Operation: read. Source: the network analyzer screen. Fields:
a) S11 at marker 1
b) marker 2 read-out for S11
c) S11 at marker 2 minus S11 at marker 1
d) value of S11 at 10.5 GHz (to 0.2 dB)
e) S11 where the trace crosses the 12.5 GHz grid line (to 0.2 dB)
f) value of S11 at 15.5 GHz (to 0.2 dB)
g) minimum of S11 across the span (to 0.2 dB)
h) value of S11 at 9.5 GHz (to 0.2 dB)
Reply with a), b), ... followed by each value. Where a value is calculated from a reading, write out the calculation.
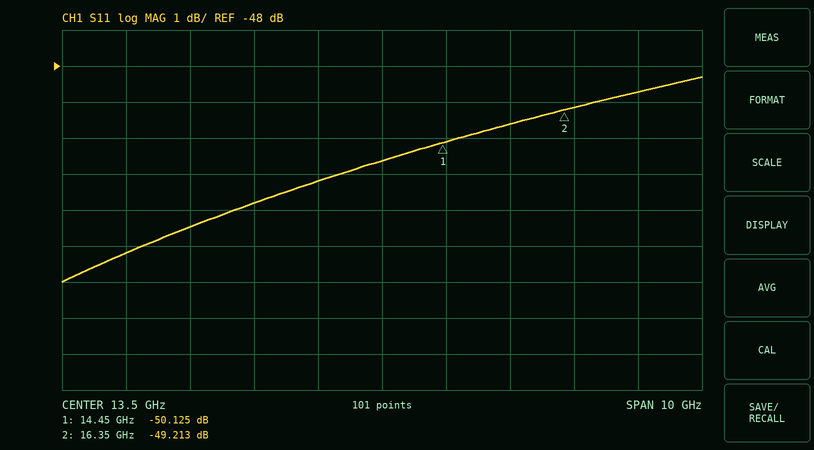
a) -50.125 dB
b) -49.213 dB
c) -49.213 − (-50.125) = 0.912 dB
d) -52.4 dB
e) -51.2 dB
f) -49.6 dB
g) -54.0 dB
h) -53.2 dB
